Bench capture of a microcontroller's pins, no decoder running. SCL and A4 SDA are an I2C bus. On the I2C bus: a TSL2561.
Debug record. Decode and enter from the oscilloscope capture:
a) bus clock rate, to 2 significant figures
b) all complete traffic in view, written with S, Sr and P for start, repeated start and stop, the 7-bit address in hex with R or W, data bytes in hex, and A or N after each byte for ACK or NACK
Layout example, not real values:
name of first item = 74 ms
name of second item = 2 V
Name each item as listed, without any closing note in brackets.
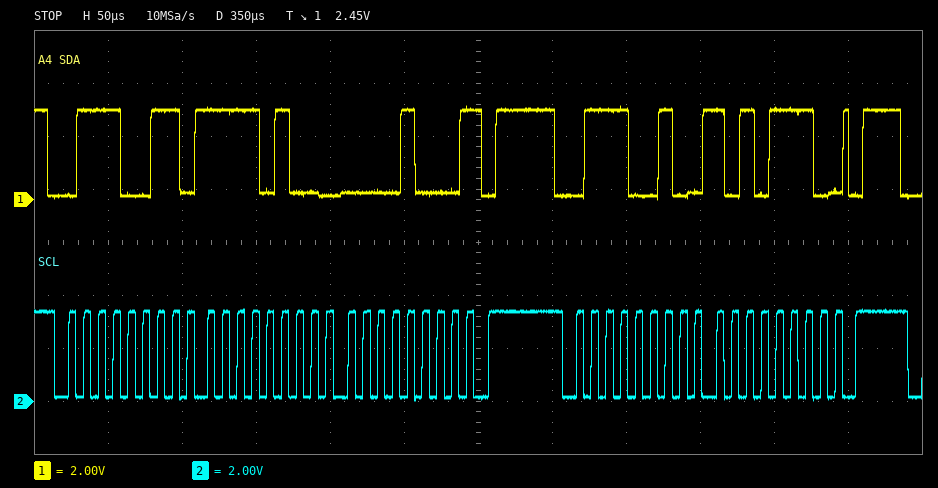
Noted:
bus clock rate, to 2 significant figures = 100 kHz
all complete traffic in view, written with S, Sr and P for start, repeated start and stop, the 7-bit address in hex with R or W, data bytes in hex, and A or N after each byte for ACK or NACK = S 39R A F4 A 08 N P S 39W A AE A P
